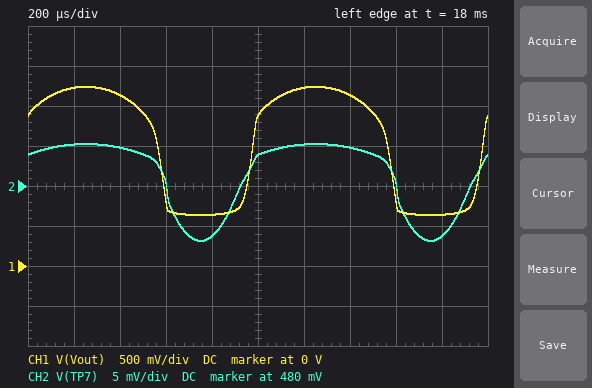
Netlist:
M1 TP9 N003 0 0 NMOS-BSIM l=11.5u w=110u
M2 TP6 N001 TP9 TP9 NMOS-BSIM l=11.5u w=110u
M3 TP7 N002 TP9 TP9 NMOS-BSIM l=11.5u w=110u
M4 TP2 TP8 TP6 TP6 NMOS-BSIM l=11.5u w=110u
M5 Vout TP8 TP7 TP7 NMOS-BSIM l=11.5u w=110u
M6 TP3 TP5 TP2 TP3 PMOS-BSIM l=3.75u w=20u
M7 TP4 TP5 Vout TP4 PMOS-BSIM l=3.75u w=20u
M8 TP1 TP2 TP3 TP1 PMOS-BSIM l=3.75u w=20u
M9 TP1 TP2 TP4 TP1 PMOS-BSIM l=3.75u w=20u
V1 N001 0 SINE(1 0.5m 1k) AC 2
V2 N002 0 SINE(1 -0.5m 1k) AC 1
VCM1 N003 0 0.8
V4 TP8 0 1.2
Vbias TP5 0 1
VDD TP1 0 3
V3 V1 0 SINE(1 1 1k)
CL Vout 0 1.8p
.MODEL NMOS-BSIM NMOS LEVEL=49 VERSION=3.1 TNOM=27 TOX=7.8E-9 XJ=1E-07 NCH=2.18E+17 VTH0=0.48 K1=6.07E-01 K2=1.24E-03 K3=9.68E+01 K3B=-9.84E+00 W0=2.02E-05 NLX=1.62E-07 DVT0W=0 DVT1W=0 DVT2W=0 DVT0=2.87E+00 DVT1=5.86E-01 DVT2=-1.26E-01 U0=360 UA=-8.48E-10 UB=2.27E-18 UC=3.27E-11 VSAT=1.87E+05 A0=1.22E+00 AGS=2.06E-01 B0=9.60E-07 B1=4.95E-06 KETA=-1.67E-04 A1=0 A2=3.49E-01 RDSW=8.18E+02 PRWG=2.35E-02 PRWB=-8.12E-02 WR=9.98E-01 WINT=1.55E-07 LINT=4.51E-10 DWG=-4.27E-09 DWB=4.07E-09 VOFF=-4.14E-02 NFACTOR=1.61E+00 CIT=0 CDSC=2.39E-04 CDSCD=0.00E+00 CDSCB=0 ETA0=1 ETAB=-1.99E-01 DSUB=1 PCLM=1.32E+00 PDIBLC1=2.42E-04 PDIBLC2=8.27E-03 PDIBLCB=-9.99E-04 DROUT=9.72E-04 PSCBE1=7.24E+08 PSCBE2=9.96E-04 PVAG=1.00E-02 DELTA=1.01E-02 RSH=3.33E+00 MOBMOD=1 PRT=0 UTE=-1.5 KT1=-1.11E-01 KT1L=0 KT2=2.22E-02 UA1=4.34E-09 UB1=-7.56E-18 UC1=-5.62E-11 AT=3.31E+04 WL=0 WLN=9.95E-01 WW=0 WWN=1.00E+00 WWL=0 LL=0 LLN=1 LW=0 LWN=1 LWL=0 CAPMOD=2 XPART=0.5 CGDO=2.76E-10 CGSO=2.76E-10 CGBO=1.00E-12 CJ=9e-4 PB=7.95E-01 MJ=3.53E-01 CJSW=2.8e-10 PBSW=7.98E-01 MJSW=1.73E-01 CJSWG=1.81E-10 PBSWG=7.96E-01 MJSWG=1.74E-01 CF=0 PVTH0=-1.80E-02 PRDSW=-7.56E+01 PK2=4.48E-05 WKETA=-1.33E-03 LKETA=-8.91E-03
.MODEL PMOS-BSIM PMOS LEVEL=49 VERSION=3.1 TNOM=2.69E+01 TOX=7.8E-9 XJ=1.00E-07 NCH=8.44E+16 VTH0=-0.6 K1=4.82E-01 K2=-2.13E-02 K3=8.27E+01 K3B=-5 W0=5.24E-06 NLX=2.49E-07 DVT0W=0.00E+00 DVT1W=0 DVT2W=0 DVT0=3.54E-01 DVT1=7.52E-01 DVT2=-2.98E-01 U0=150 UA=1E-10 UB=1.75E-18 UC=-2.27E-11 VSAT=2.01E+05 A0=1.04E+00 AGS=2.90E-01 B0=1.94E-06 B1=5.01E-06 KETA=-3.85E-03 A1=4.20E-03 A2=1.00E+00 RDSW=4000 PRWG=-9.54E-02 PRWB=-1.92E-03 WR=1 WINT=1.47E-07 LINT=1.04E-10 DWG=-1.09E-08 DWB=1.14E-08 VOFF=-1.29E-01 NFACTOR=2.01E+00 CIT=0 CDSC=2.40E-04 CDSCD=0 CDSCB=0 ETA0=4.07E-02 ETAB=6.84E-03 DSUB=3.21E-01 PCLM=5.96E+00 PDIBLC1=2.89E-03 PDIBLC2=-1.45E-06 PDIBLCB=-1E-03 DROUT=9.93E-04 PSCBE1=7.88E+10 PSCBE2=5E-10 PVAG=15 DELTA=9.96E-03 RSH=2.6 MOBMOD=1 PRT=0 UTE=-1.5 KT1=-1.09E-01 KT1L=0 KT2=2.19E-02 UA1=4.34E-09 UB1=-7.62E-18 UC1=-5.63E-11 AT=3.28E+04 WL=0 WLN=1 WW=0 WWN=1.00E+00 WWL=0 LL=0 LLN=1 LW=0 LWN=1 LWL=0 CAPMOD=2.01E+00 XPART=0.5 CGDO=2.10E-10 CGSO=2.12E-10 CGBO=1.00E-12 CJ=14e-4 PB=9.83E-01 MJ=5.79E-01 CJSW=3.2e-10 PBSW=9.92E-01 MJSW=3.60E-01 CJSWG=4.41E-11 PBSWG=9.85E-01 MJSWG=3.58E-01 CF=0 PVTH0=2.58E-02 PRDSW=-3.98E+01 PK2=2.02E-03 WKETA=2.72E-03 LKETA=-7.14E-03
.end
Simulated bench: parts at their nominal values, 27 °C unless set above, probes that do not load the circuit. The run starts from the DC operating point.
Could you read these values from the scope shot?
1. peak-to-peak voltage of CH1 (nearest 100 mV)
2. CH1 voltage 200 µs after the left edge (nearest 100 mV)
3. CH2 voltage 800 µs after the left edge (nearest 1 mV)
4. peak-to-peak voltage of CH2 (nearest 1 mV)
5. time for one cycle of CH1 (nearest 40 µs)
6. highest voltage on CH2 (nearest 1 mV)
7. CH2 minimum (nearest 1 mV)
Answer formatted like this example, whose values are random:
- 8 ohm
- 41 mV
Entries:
- 1.6 V
- 2.2 V
- 474 mV
- 12 mV
- 1.00 ms
- 485 mV
- 473 mV
